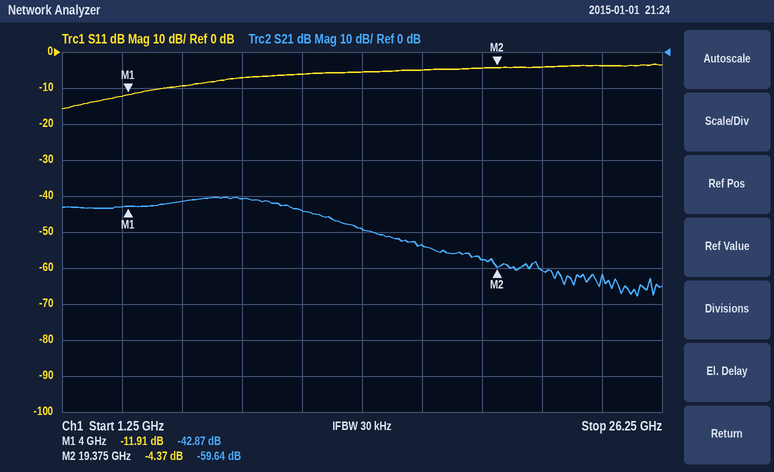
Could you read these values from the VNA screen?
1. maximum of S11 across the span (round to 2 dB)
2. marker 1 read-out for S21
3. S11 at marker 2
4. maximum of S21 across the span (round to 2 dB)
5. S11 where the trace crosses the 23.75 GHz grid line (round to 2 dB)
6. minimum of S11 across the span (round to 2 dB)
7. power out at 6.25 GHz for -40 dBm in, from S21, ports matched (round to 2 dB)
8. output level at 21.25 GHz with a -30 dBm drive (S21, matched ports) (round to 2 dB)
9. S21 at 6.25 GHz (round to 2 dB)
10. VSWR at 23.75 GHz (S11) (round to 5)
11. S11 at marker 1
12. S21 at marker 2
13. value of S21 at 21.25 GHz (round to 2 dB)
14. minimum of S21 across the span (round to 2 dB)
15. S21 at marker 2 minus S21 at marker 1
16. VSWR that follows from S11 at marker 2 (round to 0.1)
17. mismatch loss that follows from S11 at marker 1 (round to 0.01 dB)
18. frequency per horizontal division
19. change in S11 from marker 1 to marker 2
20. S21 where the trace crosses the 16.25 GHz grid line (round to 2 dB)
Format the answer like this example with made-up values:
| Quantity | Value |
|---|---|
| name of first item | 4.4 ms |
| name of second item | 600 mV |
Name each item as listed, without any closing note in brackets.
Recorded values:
| Quantity | Value |
|---|---|
| maximum of S11 across the span | -4 dB |
| marker 1 read-out for S21 | -42.87 dB |
| S11 at marker 2 | -4.37 dB |
| maximum of S21 across the span | -40 dB |
| S11 where the trace crosses the 23.75 GHz grid line | -4 dB |
| minimum of S11 across the span | -16 dB |
| power out at 6.25 GHz for -40 dBm in, from S21, ports matched | -82 dBm |
| output level at 21.25 GHz with a -30 dBm drive (S21, matched ports) | -90 dBm |
| S21 at 6.25 GHz | -42 dB |
| VSWR at 23.75 GHz (S11) | 5 |
| S11 at marker 1 | -11.91 dB |
| S21 at marker 2 | -59.64 dB |
| value of S21 at 21.25 GHz | -60 dB |
| minimum of S21 across the span | -68 dB |
| S21 at marker 2 minus S21 at marker 1 | -16.77 dB |
| VSWR that follows from S11 at marker 2 | 4.1 |
| mismatch loss that follows from S11 at marker 1 | 0.29 dB |
| frequency per horizontal division | 2.5 GHz |
| change in S11 from marker 1 to marker 2 | 7.54 dB |
| S21 where the trace crosses the 16.25 GHz grid line | -54 dB |
